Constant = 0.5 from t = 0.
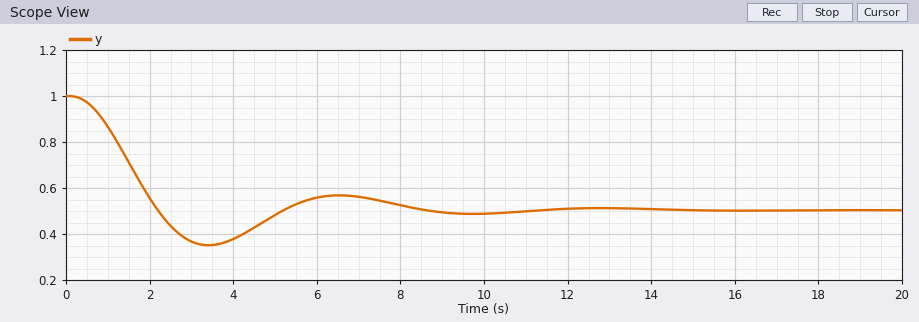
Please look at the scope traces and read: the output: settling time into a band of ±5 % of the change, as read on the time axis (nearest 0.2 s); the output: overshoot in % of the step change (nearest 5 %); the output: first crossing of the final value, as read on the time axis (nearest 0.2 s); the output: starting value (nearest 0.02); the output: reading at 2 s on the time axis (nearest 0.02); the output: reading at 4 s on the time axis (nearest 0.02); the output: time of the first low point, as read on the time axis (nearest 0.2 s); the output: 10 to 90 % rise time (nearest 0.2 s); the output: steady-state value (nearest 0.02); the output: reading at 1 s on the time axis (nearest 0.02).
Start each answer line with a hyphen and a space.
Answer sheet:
- 8.0 s
- 30 %
- 2.2 s
- 1.00
- 0.56
- 0.38
- 3.4 s
- 1.4 s
- 0.50
- 0.86
